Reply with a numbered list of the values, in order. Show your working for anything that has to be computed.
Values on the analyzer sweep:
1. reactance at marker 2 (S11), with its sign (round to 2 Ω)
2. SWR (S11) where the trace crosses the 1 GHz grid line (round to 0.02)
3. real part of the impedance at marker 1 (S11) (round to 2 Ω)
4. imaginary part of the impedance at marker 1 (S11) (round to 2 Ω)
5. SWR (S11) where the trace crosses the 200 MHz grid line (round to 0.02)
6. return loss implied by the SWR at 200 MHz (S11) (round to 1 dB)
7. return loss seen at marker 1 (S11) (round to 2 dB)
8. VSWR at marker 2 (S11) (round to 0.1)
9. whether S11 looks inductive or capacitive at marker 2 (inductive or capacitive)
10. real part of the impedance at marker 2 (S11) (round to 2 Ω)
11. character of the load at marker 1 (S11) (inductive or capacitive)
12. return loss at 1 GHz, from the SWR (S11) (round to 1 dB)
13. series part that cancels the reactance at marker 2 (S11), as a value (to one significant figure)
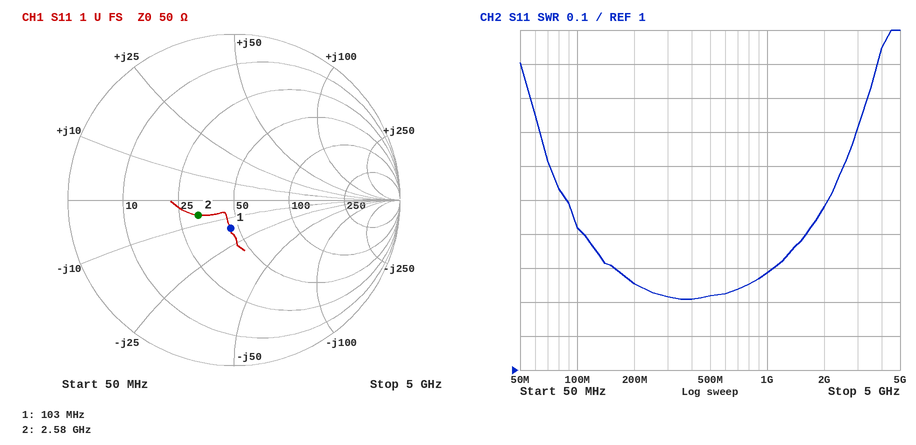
1. -6 Ω
2. 1.28
3. 46 Ω
4. -16 Ω
5. 1.26
6. −20 log10((1.26 − 1)/(1.26 + 1)) ≈ 19 dB
7. 16 dB
8. 1.6
9. capacitive
10. 32 Ω
11. capacitive
12. −20 log10((1.28 − 1)/(1.28 + 1)) ≈ 18 dB
13. L = 6 Ω/(2π × 2.58 GHz) ≈ 370 pH, so 400 pH to one significant figure
